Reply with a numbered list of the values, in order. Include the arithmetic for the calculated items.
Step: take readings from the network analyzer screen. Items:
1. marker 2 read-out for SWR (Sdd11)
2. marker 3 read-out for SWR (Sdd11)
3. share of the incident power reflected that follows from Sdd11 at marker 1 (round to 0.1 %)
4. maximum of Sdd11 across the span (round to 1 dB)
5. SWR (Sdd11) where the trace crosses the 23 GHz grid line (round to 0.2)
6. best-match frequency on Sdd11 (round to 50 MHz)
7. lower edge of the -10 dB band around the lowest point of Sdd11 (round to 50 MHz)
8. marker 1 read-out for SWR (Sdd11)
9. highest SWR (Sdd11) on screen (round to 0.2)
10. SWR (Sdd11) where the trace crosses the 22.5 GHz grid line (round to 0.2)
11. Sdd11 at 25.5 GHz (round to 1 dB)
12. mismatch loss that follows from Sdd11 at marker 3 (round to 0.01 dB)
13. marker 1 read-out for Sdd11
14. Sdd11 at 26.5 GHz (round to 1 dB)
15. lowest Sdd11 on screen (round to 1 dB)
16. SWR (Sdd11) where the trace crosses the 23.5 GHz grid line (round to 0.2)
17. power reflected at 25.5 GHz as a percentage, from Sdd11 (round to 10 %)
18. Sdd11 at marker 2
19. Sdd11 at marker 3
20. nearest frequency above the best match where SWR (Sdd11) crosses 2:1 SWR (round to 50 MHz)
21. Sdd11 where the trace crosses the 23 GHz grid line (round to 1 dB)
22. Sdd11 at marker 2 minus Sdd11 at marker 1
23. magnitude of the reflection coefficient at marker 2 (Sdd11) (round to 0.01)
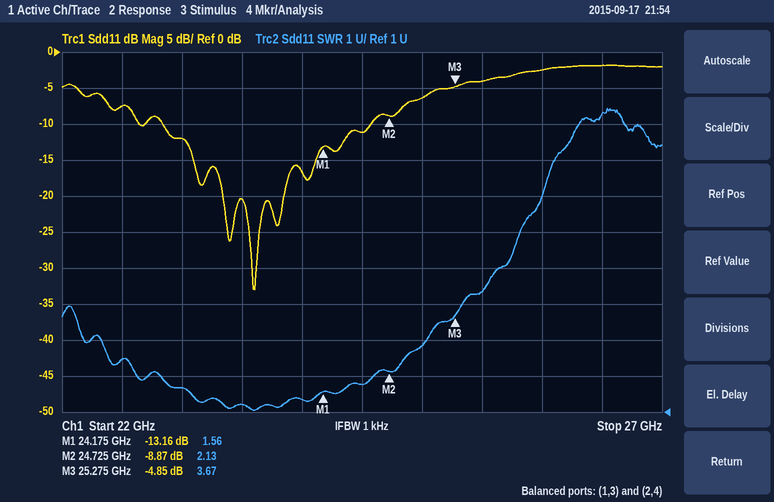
1. 2.13
2. 3.67
3. 10^(-13.16/10) ≈ 4.8 %
4. -2 dB
5. 1.6
6. 23.60 GHz
7. 22.85 GHz
8. 1.56
9. 9.4
10. 2.4
11. -4 dB
12. −10 log10(1 − 10^(-4.85/10)) ≈ 1.72 dB
13. -13.16 dB
14. -2 dB
15. -33 dB
16. 1.2
17. 10^(-4/10) ≈ 40 %
18. -8.87 dB
19. -4.85 dB
20. 24.60 GHz
21. -12 dB
22. -8.87 − (-13.16) = 4.29 dB
23. 10^(-8.87/20) ≈ 0.36
